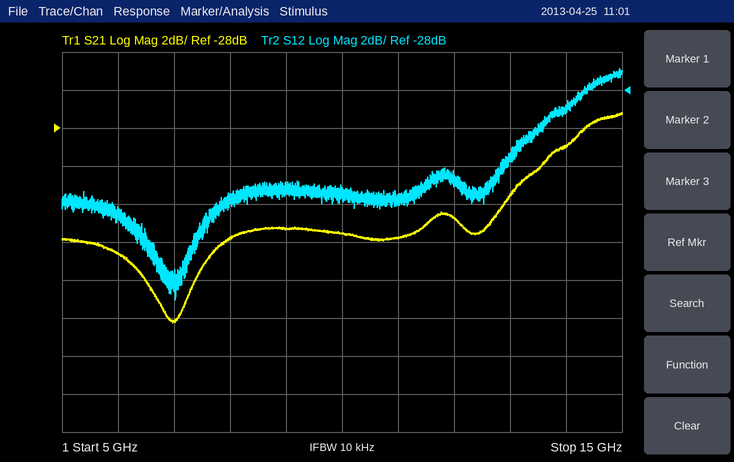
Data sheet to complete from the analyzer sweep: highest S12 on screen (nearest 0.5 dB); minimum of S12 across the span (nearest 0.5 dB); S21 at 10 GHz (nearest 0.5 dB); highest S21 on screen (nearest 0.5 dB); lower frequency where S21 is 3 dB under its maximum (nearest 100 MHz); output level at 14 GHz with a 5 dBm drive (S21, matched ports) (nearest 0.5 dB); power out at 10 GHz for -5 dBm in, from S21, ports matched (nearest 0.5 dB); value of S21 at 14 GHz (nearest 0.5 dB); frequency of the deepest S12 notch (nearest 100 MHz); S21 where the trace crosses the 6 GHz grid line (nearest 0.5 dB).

-27.0 dB
-39.0 dB
-33.5 dB
-27.0 dB
13.5 GHz
-24.0 dBm
-38.5 dBm
-29.0 dB
7.0 GHz
-34.5 dB
